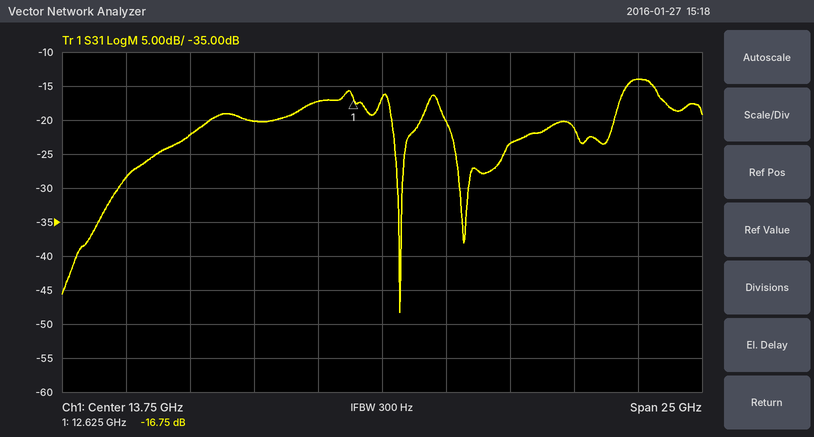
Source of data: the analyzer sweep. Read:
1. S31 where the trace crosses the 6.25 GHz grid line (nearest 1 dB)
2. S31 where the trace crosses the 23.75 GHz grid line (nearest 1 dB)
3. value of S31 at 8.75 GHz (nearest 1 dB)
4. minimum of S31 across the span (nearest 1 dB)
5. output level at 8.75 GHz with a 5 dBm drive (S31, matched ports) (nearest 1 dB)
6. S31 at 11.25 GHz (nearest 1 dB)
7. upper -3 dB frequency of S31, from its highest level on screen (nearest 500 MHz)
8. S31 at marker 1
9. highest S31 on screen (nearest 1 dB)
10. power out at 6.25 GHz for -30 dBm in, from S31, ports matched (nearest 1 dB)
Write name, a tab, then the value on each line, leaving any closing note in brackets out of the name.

S31 where the trace crosses the 6.25 GHz grid line	-22 dB
S31 where the trace crosses the 23.75 GHz grid line	-14 dB
value of S31 at 8.75 GHz	-20 dB
minimum of S31 across the span	-48 dB
output level at 8.75 GHz with a 5 dBm drive (S31, matched ports)	-15 dBm
S31 at 11.25 GHz	-17 dB
upper -3 dB frequency of S31, from its highest level on screen	24.5 GHz
S31 at marker 1	-16.75 dB
highest S31 on screen	-14 dB
power out at 6.25 GHz for -30 dBm in, from S31, ports matched	-52 dBm
